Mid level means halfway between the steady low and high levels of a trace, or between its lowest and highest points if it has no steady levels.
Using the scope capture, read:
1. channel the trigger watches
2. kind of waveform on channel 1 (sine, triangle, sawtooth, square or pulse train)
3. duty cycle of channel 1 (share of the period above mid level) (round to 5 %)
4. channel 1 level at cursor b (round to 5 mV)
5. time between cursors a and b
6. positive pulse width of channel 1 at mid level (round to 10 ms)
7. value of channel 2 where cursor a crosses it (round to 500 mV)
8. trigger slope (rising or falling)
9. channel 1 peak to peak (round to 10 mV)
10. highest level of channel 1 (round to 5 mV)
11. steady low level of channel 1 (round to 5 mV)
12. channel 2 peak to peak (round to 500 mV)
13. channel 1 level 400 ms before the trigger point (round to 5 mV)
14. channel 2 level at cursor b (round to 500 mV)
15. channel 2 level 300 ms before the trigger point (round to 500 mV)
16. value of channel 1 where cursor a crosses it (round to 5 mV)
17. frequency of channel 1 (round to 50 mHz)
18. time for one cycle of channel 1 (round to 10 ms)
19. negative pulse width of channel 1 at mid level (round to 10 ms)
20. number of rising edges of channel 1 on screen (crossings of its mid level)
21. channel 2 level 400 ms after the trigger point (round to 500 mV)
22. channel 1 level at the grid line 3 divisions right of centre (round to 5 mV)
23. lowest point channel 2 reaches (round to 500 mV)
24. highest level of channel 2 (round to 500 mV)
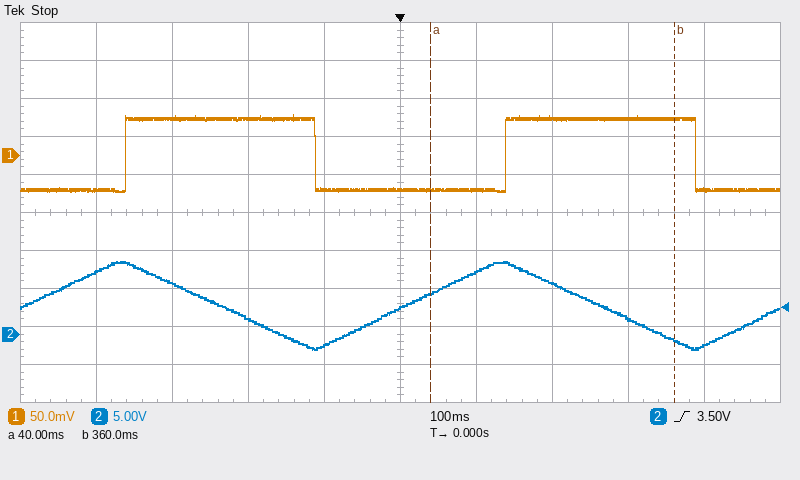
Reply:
channel 2
square
50 %
50 mV
320 ms
250 ms
5.5 V
rising
100 mV
55 mV
-45 mV
11.5 V
-45 mV
-1.0 V
6.5 V
-45 mV
2.00 Hz
500 ms
250 ms
2
-1.5 V
50 mV
-2.0 V
9.5 V
